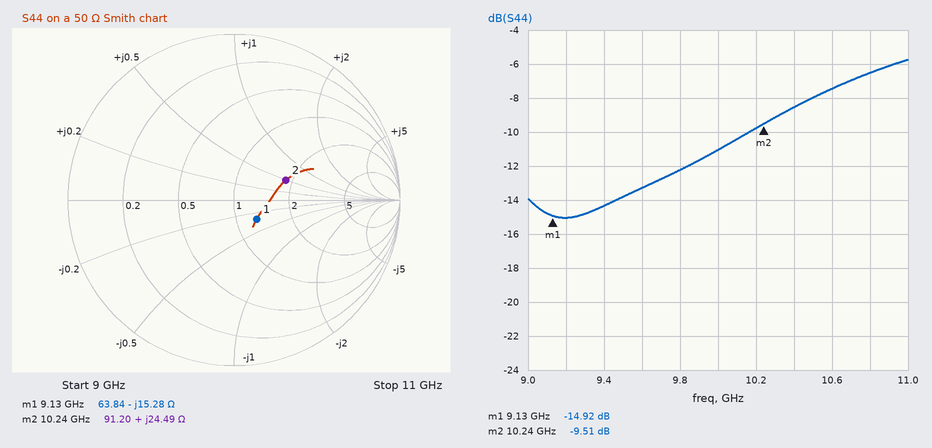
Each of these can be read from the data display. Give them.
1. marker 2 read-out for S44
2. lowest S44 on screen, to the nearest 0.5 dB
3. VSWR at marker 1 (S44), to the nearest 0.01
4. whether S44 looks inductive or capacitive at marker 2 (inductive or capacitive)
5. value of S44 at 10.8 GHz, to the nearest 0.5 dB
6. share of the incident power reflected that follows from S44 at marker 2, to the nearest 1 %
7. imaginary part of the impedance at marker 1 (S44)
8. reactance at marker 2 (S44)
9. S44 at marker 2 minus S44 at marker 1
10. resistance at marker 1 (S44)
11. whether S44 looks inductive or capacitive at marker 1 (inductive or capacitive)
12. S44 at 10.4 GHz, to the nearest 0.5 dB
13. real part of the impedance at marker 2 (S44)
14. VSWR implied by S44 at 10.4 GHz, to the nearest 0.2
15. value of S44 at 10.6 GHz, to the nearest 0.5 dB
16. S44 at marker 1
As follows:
-9.51 dB
-15.0 dB
1.44
inductive
-6.5 dB
11 %
-15.28 Ω
+24.49 Ω
5.41 dB
63.84 Ω
capacitive
-8.5 dB
91.20 Ω
2.2
-7.5 dB
-14.92 dB
